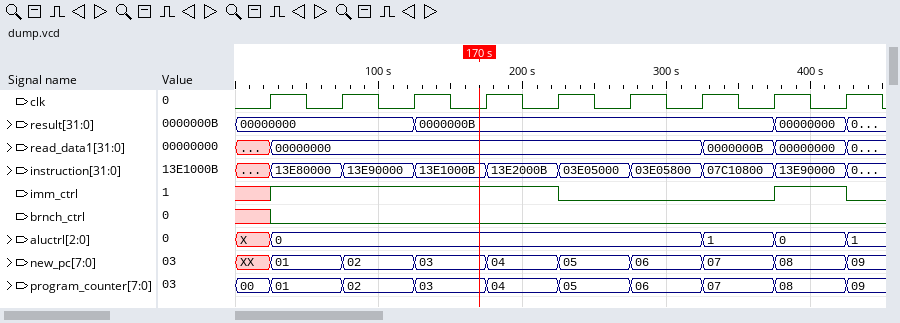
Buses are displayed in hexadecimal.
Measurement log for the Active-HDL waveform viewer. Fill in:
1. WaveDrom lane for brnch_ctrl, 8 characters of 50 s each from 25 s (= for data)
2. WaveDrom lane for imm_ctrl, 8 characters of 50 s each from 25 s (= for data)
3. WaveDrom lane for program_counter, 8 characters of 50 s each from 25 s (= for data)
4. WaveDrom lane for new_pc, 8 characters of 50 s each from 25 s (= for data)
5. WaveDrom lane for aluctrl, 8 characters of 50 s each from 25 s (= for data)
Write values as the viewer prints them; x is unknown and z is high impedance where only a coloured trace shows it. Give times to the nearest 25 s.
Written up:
{name: 'brnch_ctrl', wave: '0.......'}
{name: 'imm_ctrl', wave: '1...0..1'}
{name: 'program_counter', wave: '========', data: '01 02 03 04 05 06 07 08'}
{name: 'new_pc', wave: '========', data: '01 02 03 04 05 06 07 08'}
{name: 'aluctrl', wave: '=.....==', data: '0 1 0'}
